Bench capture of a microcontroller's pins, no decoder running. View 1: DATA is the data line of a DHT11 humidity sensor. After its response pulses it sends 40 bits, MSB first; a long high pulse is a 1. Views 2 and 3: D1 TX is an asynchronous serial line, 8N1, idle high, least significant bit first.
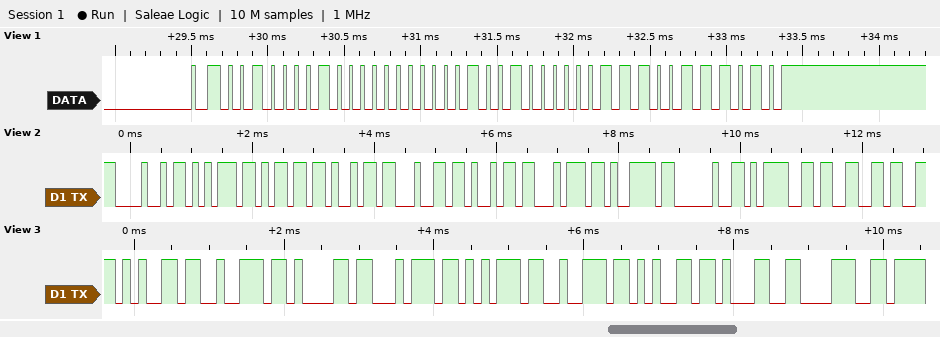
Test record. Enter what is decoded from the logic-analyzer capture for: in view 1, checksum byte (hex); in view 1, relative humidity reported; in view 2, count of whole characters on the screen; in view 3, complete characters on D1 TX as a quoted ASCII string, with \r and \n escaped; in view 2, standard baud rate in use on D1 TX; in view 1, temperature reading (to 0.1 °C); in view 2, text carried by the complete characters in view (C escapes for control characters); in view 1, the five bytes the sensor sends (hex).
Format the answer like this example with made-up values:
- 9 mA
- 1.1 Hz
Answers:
- 0x3A
- 33 %
- 11
- "erature18"
- 9600 baud
- 18.7 °C
- "Humidity =3"
- 21 00 12 07 3A
